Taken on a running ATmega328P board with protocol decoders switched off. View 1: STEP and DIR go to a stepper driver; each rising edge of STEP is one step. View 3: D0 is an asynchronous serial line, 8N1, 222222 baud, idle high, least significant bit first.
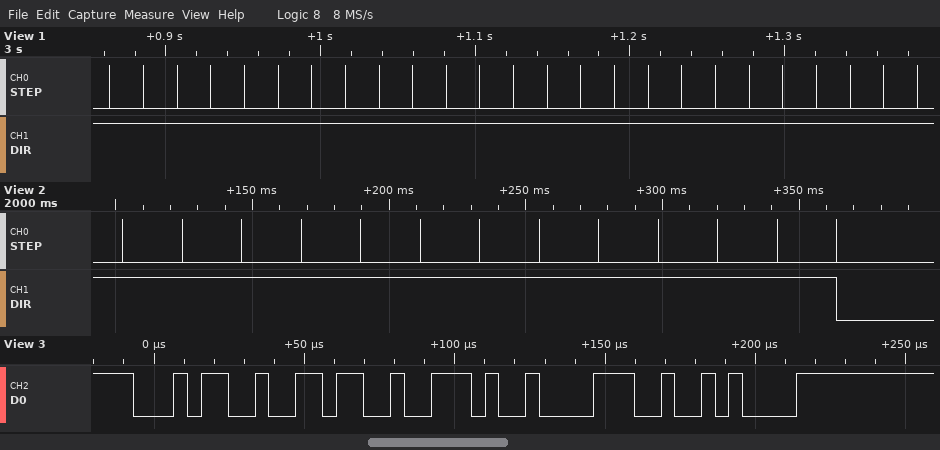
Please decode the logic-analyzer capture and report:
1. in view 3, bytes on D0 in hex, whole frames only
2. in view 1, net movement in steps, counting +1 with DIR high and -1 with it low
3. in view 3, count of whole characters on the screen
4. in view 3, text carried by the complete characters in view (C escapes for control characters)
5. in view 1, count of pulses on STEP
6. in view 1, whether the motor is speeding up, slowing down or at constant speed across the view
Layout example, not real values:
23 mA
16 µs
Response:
34 36 2E 38 0A
+25
5
"46.8\n"
25
constant speed
